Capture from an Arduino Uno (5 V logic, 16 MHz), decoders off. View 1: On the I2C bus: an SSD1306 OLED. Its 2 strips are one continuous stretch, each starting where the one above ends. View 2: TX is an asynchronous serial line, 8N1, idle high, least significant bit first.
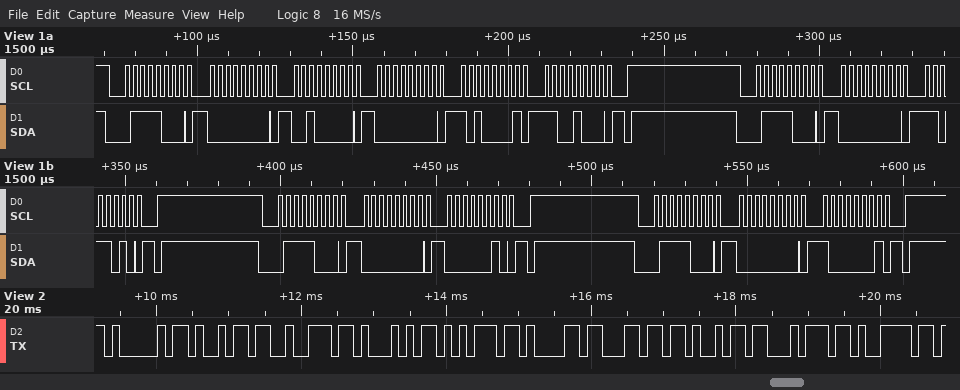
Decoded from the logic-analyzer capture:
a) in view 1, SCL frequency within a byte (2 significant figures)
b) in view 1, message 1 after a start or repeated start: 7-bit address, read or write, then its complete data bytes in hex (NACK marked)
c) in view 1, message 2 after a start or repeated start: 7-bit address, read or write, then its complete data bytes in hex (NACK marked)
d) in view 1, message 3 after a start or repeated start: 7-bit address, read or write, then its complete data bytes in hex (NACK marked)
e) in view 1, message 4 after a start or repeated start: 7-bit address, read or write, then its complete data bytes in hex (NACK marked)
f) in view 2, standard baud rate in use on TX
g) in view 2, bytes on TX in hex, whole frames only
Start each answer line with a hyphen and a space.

- 400 kHz
- 0x3C write: 00 20 00 A1 C8
- 0x3C write: 00 DA
- 0x3C write: 00 02
- 0x3C write: 00 81
- 9600 baud
- 0x41 0x69 0x72 0x51 0x75 0x61 0x6C 0x69 0x74 0x79
